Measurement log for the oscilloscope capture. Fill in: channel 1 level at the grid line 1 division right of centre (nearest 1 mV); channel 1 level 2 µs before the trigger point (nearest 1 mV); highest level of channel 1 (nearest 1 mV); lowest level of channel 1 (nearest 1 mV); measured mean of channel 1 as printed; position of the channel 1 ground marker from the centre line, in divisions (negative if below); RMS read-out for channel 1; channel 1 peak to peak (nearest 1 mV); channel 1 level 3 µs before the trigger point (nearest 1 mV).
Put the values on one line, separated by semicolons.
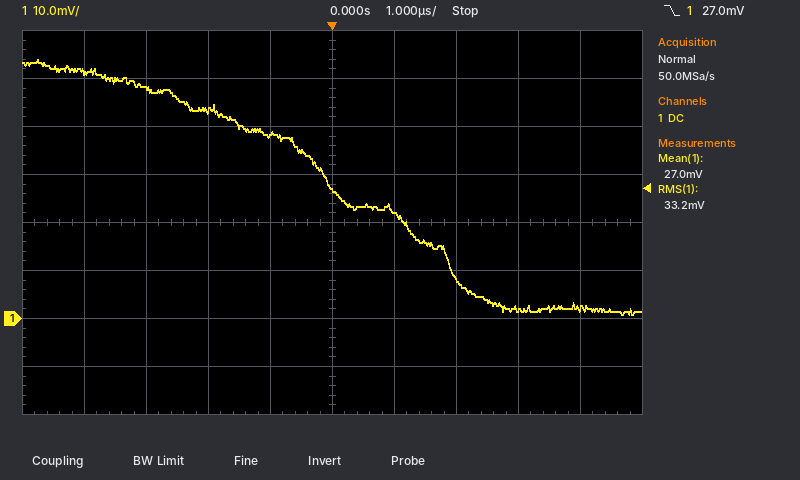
22 mV; 43 mV; 54 mV; 1 mV; 27.0 mV; -2.0 div; 33.2 mV; 53 mV; 48 mV
